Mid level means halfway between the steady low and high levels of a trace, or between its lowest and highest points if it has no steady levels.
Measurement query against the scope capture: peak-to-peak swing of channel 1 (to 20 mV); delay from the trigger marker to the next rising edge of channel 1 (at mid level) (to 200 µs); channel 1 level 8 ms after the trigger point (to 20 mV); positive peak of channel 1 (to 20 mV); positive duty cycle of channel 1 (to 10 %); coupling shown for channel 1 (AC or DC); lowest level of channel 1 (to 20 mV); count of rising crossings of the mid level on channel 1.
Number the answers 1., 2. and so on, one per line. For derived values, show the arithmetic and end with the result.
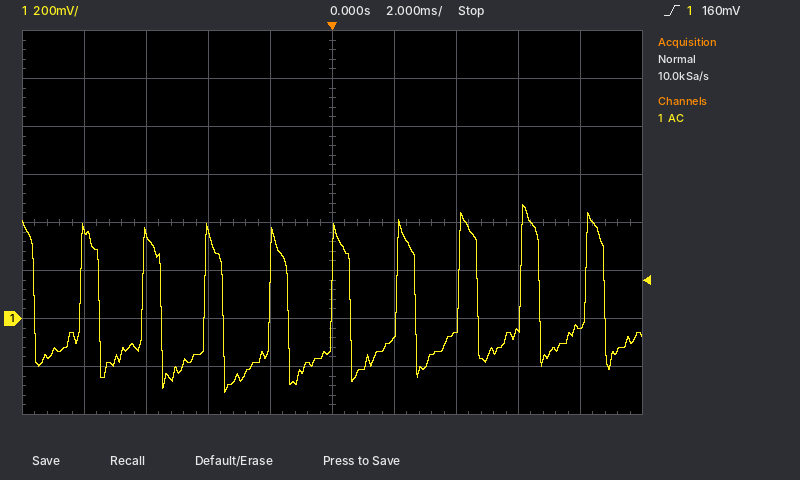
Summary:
1. 480 mV − (-300 mV) = 780 mV
2. 2.0 ms
3. -40 mV
4. 480 mV
5. 30 %
6. AC
7. -300 mV
8. 9
